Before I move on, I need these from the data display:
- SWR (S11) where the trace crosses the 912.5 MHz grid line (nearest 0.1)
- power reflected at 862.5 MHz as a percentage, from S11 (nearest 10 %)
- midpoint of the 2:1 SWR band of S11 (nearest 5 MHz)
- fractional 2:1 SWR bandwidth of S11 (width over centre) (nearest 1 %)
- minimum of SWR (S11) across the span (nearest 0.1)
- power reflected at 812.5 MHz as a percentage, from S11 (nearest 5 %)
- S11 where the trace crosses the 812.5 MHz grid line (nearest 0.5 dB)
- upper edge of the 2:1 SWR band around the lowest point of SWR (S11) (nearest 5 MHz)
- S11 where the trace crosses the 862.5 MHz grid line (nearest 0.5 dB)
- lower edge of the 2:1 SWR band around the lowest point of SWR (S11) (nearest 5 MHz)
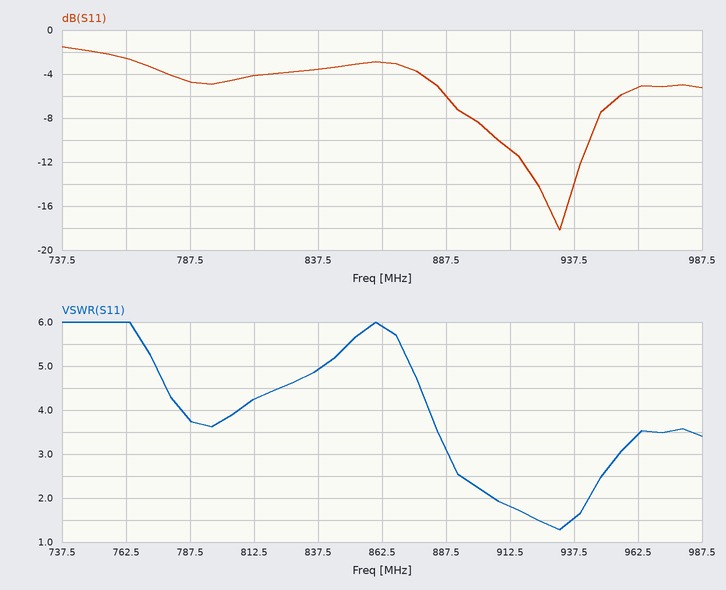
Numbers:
1.8
50 %
925 MHz
4 %
1.3
40 %
-4.0 dB
945 MHz
-3.0 dB
905 MHz
